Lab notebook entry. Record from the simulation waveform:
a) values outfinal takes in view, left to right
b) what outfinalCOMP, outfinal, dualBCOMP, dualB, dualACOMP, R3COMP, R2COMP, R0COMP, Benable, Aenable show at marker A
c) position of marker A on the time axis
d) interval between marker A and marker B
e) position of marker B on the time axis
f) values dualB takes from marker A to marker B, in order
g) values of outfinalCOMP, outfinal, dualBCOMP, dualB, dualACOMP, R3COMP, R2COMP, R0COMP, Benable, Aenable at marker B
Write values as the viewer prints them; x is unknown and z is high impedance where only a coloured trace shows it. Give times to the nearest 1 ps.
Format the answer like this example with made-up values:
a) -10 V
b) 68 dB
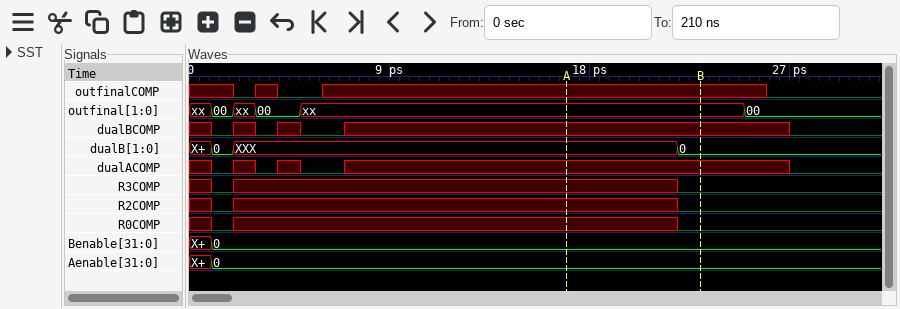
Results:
a) xx, 00, xx, 00, xx, 00
b) outfinalCOMP=x, outfinal=xx, dualBCOMP=x, dualB=XXX, dualACOMP=x, R3COMP=x, R2COMP=x, R0COMP=x, Benable=0, Aenable=0
c) 17 ps
d) 6 ps
e) 23 ps
f) XXX, 0
g) outfinalCOMP=x, outfinal=xx, dualBCOMP=x, dualB=0, dualACOMP=x, R3COMP=0, R2COMP=0, R0COMP=0, Benable=0, Aenable=0
